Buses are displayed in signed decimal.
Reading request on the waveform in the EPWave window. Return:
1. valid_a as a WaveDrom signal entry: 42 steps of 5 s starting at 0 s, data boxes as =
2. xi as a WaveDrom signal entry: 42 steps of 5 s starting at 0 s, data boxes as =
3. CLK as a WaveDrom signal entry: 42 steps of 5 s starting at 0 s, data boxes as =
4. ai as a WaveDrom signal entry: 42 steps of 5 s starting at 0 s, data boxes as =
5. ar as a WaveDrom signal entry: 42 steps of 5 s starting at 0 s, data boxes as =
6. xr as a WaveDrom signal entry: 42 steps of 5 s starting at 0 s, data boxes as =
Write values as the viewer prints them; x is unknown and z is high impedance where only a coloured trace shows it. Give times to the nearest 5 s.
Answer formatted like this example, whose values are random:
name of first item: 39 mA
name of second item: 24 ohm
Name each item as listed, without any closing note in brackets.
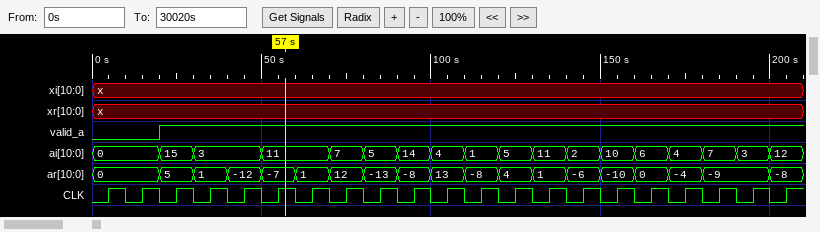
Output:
valid_a as a WaveDrom signal entry: 42 steps of 5 s starting at 0 s, data boxes as =: {name: 'valid_a', wave: '0...1.....................................'}
xi as a WaveDrom signal entry: 42 steps of 5 s starting at 0 s, data boxes as =: {name: 'xi', wave: 'x.........................................'}
CLK as a WaveDrom signal entry: 42 steps of 5 s starting at 0 s, data boxes as =: {name: 'CLK', wave: '010101010101010101010101010101010101010101'}
ai as a WaveDrom signal entry: 42 steps of 5 s starting at 0 s, data boxes as =: {name: 'ai', wave: '=...=.=...=...=.=.=.=.=.=.=.=.=.=.=.=.=.=.', data: '0 15 3 11 7 5 14 4 1 5 11 2 10 6 4 7 3 12'}
ar as a WaveDrom signal entry: 42 steps of 5 s starting at 0 s, data boxes as =: {name: 'ar', wave: '=...=.=.=.=.=.=.=.=.=.=.=.=.=.=.=.=.=...=.', data: '0 5 1 -12 -7 1 12 -13 -8 13 -8 4 1 -6 -10 0 -4 -9 -8'}
xr as a WaveDrom signal entry: 42 steps of 5 s starting at 0 s, data boxes as =: {name: 'xr', wave: 'x.........................................'}
